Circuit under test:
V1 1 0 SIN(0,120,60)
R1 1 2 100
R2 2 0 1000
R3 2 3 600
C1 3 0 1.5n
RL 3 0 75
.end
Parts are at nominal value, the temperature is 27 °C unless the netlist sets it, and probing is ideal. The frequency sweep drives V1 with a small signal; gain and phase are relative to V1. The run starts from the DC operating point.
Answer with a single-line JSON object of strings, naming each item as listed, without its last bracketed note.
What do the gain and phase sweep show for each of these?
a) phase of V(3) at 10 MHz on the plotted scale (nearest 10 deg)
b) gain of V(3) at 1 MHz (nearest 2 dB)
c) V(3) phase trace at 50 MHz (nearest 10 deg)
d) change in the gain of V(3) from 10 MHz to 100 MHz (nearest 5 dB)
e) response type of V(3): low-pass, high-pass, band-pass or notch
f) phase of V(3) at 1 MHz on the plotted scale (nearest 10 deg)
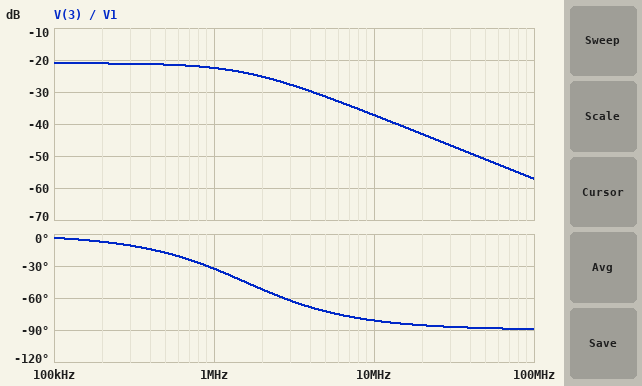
{"phase of V(3) at 10 MHz on the plotted scale": "-80 deg", "gain of V(3) at 1 MHz": "-22 dB", "V(3) phase trace at 50 MHz": "-90 deg", "change in the gain of V(3) from 10 MHz to 100 MHz": "-20 dB", "response type of V(3): low-pass, high-pass, band-pass or notch": "low-pass", "phase of V(3) at 1 MHz on the plotted scale": "-30 deg"}
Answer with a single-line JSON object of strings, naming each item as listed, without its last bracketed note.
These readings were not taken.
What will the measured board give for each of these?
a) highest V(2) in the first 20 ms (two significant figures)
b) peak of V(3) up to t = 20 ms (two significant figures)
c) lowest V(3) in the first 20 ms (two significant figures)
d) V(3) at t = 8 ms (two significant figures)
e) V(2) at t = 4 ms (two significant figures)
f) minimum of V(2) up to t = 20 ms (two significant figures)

{"highest V(2) in the first 20 ms": "96 V", "peak of V(3) up to t = 20 ms": "11 V", "lowest V(3) in the first 20 ms": "-11 V", "V(3) at t = 8 ms": "1.3 V", "V(2) at t = 4 ms": "96 V", "minimum of V(2) up to t = 20 ms": "-96 V"}
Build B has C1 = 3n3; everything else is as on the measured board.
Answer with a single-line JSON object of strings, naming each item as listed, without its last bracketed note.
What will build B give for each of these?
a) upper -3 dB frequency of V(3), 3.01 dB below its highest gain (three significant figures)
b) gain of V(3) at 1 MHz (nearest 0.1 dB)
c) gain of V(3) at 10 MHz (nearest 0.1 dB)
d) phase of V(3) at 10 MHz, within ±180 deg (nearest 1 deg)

{"upper -3 dB frequency of V(3), 3.01 dB below its highest gain": "713 kHz", "gain of V(3) at 1 MHz": "-25.7 dB", "gain of V(3) at 10 MHz": "-44.0 dB", "phase of V(3) at 10 MHz, within ±180 deg": "-86 deg"}
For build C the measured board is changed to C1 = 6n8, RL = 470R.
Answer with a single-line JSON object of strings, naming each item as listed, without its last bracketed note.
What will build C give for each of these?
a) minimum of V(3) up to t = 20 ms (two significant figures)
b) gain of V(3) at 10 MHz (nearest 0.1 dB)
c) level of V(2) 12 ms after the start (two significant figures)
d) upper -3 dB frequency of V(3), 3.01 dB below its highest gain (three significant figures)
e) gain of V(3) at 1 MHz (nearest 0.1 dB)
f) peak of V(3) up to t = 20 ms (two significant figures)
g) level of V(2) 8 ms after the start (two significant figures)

{"minimum of V(3) up to t = 20 ms": "-44 V", "gain of V(3) at 10 MHz": "-50.2 dB", "level of V(2) 12 ms after the start": "-99 V", "upper -3 dB frequency of V(3), 3.01 dB below its highest gain": "83.7 kHz", "gain of V(3) at 1 MHz": "-30.3 dB", "peak of V(3) up to t = 20 ms": "44 V", "level of V(2) 8 ms after the start": "13 V"}
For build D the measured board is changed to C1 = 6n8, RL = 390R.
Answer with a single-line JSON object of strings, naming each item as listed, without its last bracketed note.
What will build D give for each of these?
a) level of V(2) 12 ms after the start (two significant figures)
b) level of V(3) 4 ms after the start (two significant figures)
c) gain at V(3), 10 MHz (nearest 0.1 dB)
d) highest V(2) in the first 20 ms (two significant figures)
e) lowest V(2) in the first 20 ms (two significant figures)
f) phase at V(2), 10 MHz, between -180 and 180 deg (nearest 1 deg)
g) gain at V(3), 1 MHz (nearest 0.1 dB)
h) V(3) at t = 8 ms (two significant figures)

{"level of V(2) 12 ms after the start": "-98 V", "level of V(3) 4 ms after the start": "39 V", "gain at V(3), 10 MHz": "-50.2 dB", "highest V(2) in the first 20 ms": "100 V", "lowest V(2) in the first 20 ms": "-100 V", "phase at V(2), 10 MHz, between -180 and 180 deg": "0 deg", "gain at V(3), 1 MHz": "-30.3 dB", "V(3) at t = 8 ms": "5.0 V"}
